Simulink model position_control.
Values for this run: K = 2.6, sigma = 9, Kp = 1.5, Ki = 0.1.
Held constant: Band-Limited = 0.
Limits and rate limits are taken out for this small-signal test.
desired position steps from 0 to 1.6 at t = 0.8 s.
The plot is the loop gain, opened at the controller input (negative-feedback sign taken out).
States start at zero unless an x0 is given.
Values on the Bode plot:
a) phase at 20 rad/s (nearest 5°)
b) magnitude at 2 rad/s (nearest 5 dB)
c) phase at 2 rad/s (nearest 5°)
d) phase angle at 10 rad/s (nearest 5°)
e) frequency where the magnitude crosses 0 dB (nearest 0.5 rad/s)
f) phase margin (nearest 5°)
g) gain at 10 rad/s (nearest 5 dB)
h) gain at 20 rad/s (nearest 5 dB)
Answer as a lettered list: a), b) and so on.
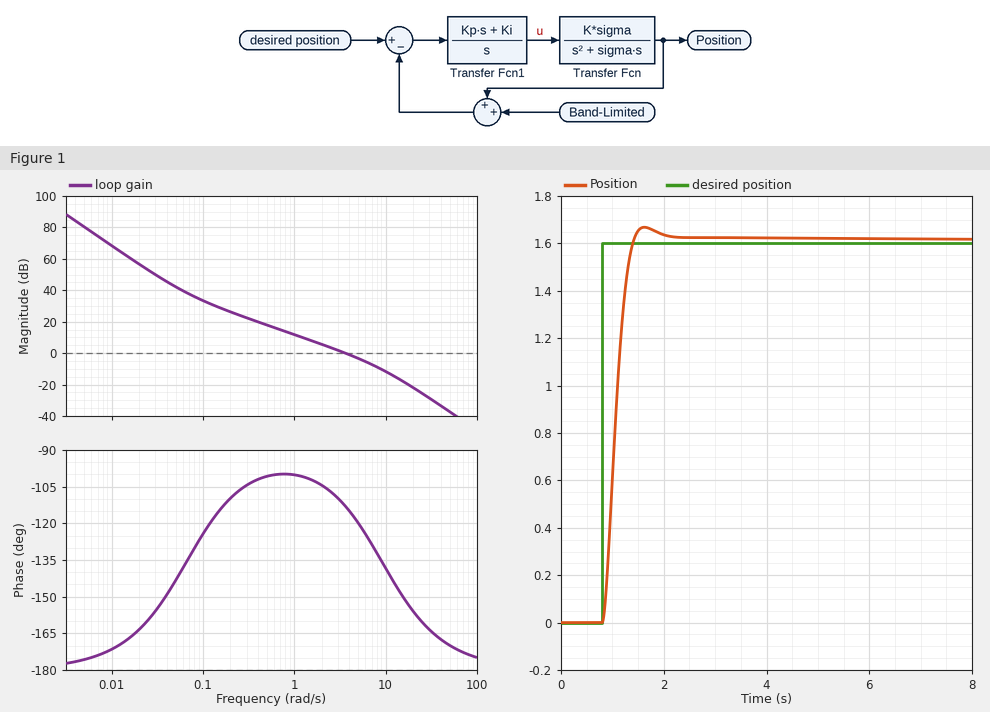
a) -155°
b) 5 dB
c) -105°
d) -140°
e) 3.5 rad/s
f) 65°
g) -10 dB
h) -20 dB
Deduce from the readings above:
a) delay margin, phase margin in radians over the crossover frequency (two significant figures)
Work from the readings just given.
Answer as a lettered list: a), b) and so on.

a) 0.32 s
